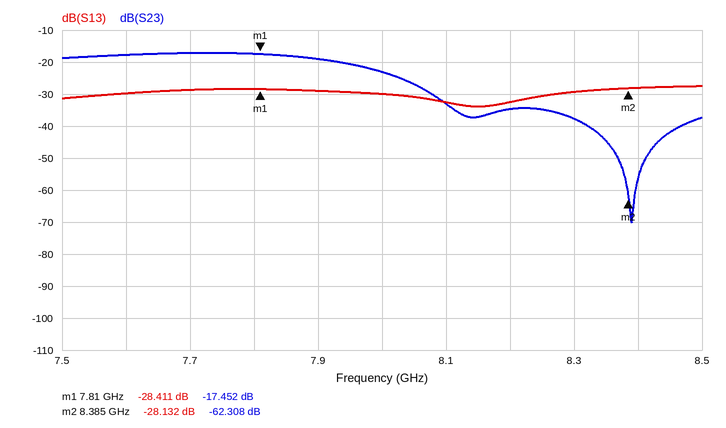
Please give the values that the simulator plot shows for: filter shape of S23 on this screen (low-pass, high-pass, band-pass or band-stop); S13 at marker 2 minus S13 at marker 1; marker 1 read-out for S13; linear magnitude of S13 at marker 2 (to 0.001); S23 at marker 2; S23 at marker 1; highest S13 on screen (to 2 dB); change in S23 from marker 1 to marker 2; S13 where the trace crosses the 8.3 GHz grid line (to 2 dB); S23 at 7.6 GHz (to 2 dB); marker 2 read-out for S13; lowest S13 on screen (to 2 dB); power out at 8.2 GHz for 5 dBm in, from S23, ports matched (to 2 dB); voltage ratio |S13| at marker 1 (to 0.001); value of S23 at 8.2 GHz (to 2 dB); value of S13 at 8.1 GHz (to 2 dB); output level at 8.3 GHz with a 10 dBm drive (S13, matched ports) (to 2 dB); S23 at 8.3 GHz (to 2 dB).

low-pass
0.279 dB
-28.411 dB
0.039
-62.308 dB
-17.452 dB
-28 dB
-44.856 dB
-30 dB
-18 dB
-28.132 dB
-34 dB
-30 dBm
0.038
-34 dB
-32 dB
-20 dBm
-38 dB
